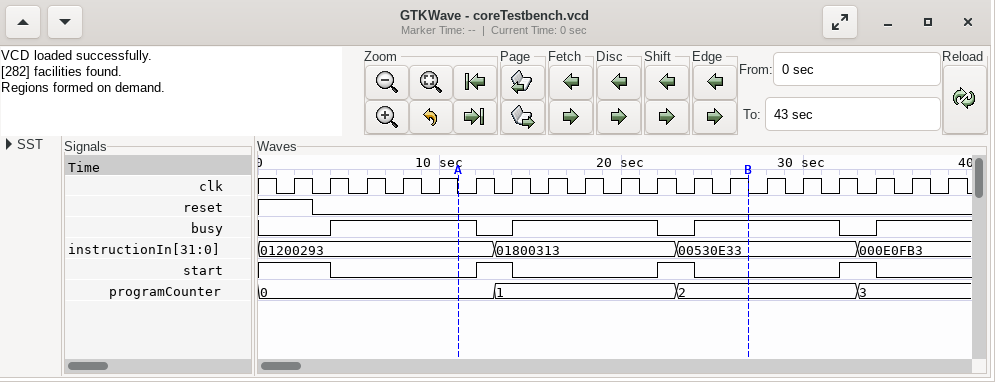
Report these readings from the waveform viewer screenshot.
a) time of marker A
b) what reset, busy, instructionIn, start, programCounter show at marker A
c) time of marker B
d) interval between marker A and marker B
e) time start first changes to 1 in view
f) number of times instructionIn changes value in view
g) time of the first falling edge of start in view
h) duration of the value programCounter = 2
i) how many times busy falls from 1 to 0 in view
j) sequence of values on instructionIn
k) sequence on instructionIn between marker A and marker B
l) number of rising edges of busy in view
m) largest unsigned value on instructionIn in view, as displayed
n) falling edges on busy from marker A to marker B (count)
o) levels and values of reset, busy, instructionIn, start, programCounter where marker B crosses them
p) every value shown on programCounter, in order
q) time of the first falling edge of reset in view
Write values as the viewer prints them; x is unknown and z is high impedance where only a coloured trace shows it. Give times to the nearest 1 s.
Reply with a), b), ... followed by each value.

a) 11 s
b) reset=0, busy=1, instructionIn=01200293, start=0, programCounter=0
c) 27 s
d) 16 s
e) 12 s
f) 3
g) 4 s
h) 10 s
i) 3
j) 01200293, 01800313, 00530E33, 000E0FB3
k) 01200293, 01800313, 00530E33
l) 4
m) 01800313
n) 2
o) reset=0, busy=1, instructionIn=00530E33, start=0, programCounter=2
p) 0, 1, 2, 3
q) 3 s
